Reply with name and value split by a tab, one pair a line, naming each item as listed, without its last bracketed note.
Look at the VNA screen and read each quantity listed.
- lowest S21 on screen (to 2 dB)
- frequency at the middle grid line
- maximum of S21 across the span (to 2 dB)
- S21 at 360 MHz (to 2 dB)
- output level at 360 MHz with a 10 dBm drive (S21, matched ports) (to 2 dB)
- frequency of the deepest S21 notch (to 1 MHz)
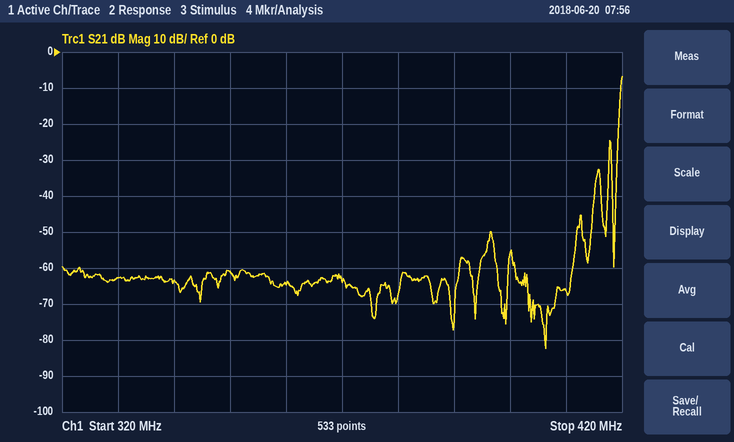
lowest S21 on screen	-82 dB
frequency at the middle grid line	370 MHz
maximum of S21 across the span	-6 dB
S21 at 360 MHz	-64 dB
output level at 360 MHz with a 10 dBm drive (S21, matched ports)	-54 dBm
frequency of the deepest S21 notch	406 MHz
